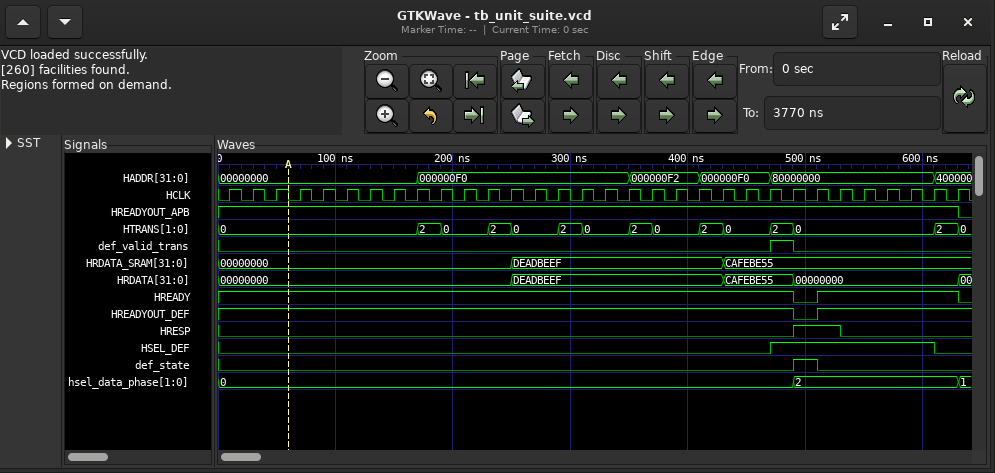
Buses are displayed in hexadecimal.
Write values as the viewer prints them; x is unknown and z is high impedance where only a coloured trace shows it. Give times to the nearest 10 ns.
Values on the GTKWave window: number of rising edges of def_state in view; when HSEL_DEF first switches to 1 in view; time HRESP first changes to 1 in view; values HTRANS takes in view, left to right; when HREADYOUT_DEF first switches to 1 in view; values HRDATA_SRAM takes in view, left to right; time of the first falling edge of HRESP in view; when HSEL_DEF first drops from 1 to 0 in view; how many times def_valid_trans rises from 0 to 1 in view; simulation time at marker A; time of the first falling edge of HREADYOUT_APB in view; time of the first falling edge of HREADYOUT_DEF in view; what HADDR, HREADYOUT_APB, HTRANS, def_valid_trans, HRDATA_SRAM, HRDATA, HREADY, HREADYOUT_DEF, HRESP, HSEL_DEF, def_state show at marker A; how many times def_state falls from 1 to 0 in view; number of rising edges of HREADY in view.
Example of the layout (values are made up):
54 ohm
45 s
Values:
1
470 ns
490 ns
0, 2, 0, 2, 0, 2, 0, 2, 0, 2, 0, 2, 0, 2, 0
510 ns
00000000, DEADBEEF, CAFEBE55
530 ns
610 ns
1
60 ns
630 ns
490 ns
HADDR=00000000, HREADYOUT_APB=1, HTRANS=0, def_valid_trans=0, HRDATA_SRAM=00000000, HRDATA=00000000, HREADY=1, HREADYOUT_DEF=1, HRESP=0, HSEL_DEF=0, def_state=0
1
1
